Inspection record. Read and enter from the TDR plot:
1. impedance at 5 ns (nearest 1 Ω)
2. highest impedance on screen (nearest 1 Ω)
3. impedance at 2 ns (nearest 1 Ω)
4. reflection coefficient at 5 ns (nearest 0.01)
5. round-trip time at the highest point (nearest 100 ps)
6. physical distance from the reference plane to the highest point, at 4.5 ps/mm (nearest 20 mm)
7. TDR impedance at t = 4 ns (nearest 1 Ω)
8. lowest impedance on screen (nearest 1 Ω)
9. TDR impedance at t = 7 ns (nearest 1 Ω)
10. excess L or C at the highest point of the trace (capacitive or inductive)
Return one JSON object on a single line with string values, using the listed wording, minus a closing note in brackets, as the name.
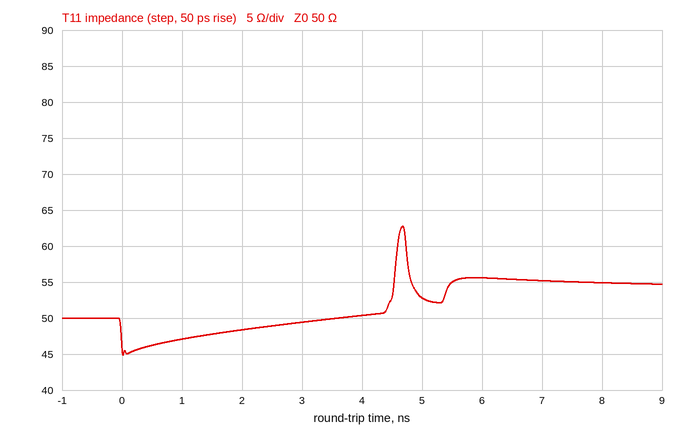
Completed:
{"impedance at 5 ns": "53 Ω", "highest impedance on screen": "63 Ω", "impedance at 2 ns": "48 Ω", "reflection coefficient at 5 ns": "+0.03", "round-trip time at the highest point": "4.7 ns", "physical distance from the reference plane to the highest point, at 4.5 ps/mm": "520 mm", "TDR impedance at t = 4 ns": "50 Ω", "lowest impedance on screen": "45 Ω", "TDR impedance at t = 7 ns": "55 Ω", "excess L or C at the highest point of the trace": "inductive"}
